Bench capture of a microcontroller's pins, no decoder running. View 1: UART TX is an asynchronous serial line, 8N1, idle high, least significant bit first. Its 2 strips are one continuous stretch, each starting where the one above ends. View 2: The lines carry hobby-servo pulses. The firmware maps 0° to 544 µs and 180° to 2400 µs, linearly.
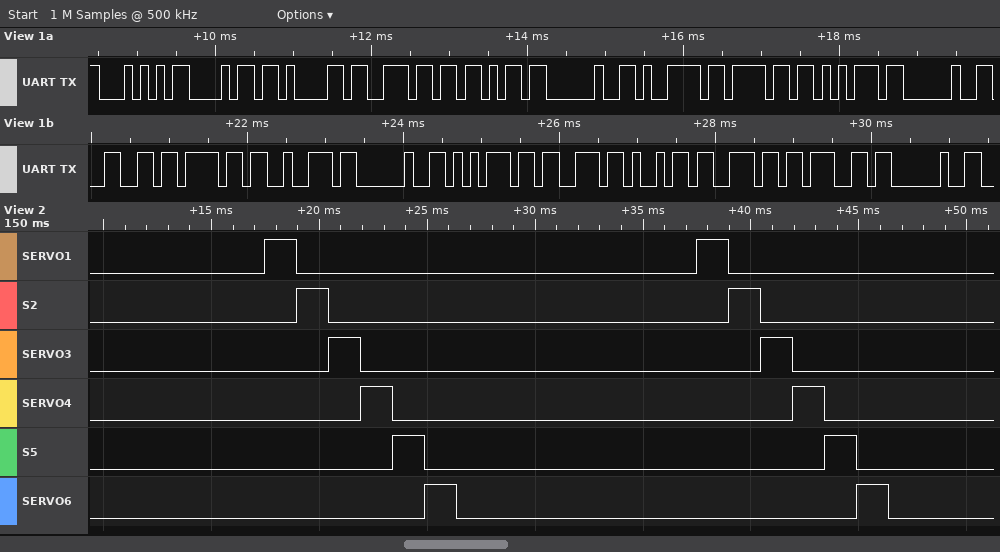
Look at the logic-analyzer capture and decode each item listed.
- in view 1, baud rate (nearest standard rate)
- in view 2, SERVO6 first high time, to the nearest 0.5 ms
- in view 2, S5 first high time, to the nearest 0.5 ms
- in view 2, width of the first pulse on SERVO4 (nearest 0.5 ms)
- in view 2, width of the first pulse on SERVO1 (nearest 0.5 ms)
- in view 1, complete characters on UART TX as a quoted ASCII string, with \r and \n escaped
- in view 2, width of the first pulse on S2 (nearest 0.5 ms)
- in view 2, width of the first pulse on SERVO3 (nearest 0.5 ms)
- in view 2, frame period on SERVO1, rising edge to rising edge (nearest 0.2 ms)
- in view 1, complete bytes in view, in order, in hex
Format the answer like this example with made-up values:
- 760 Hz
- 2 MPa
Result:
- 9600 baud
- 1.5 ms
- 1.5 ms
- 1.5 ms
- 1.5 ms
- "Thank you for using "
- 1.5 ms
- 1.5 ms
- 20.0 ms
- 0x54 0x68 0x61 0x6E 0x6B 0x20 0x79 0x6F 0x75 0x20 0x66 0x6F 0x72 0x20 0x75 0x73 0x69 0x6E 0x67 0x20
